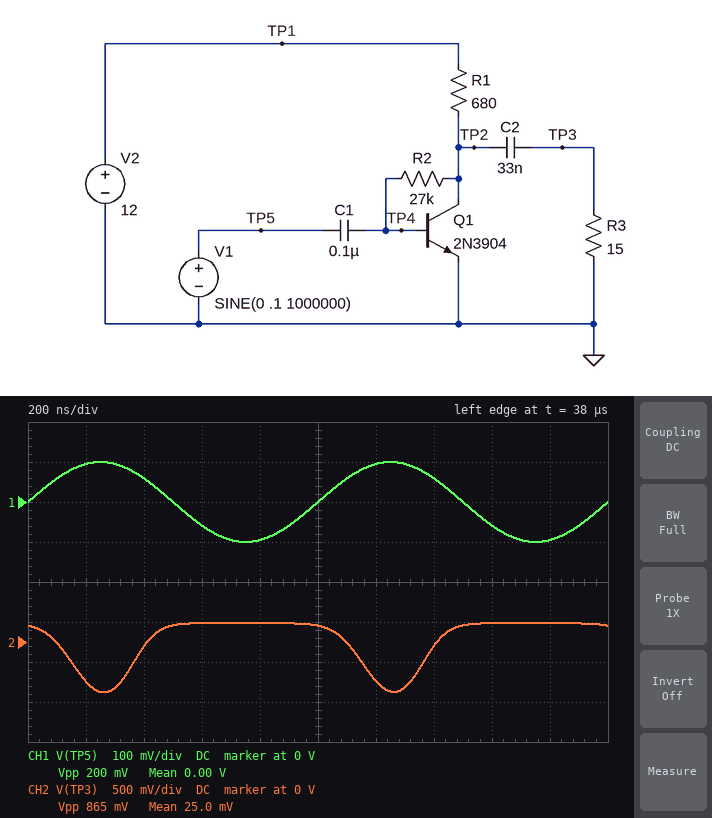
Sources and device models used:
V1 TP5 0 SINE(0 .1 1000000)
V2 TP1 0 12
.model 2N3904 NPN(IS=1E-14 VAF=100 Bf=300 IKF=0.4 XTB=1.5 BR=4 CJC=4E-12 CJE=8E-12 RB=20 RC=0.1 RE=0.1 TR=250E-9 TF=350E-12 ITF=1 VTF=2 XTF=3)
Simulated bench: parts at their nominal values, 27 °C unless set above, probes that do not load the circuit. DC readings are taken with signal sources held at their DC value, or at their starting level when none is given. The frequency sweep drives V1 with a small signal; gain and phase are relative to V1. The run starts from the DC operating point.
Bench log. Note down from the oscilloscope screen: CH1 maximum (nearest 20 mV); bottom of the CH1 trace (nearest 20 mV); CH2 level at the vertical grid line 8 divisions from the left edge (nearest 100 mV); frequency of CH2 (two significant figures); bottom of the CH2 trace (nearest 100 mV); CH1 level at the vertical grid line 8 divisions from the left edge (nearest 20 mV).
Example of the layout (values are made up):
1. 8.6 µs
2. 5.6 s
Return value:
1. 100 mV
2. -100 mV
3. 200 mV
4. 1.0 MHz
5. -600 mV
6. -60 mV
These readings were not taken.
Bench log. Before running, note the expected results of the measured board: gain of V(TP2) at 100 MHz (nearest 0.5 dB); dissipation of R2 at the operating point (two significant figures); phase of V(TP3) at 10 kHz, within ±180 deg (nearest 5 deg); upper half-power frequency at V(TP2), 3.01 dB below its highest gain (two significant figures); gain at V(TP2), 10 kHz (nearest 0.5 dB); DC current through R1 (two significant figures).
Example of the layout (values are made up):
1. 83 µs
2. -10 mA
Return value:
1. 8.0 dB
2. 66 µW
3. -60 deg
4. 19 kHz
5. 45.5 dB
6. 15 mA
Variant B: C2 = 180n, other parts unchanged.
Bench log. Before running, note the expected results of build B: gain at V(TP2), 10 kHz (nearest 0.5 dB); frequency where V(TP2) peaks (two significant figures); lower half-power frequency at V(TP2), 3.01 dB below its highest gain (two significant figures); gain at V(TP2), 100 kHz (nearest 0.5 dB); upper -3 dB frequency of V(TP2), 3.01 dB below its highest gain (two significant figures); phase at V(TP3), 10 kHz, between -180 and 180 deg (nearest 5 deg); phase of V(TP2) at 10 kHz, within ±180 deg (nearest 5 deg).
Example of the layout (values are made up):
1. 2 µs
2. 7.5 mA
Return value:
1. 34.0 dB
2. 5.4 kHz
3. 3.6 kHz
4. 18.5 dB
5. 8.3 kHz
6. -145 deg
7. 135 deg
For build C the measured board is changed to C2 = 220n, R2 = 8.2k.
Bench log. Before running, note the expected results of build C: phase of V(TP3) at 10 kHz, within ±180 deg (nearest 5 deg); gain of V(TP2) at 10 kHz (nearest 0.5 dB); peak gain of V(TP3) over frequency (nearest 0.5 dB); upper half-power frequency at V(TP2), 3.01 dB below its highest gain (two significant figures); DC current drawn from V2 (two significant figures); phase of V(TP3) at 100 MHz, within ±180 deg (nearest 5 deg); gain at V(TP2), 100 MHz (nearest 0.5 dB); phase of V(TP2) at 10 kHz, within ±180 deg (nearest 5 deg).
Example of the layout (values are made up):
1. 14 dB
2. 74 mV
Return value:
1. -110 deg
2. 35.5 dB
3. 21.5 dB
4. 12 kHz
5. 16 mA
6. 105 deg
7. 8.0 dB
8. 170 deg
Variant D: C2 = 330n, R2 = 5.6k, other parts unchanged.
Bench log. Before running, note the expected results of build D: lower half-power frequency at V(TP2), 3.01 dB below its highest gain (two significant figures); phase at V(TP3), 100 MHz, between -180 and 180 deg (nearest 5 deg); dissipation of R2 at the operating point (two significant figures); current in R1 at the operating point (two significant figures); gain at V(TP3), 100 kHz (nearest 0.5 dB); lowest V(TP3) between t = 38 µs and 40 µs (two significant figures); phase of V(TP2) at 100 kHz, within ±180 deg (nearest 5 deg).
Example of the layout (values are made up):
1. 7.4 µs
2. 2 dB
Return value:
1. 6.1 kHz
2. 105 deg
3. 17 µW
4. 16 mA
5. 18.0 dB
6. -440 mV
7. 165 deg
